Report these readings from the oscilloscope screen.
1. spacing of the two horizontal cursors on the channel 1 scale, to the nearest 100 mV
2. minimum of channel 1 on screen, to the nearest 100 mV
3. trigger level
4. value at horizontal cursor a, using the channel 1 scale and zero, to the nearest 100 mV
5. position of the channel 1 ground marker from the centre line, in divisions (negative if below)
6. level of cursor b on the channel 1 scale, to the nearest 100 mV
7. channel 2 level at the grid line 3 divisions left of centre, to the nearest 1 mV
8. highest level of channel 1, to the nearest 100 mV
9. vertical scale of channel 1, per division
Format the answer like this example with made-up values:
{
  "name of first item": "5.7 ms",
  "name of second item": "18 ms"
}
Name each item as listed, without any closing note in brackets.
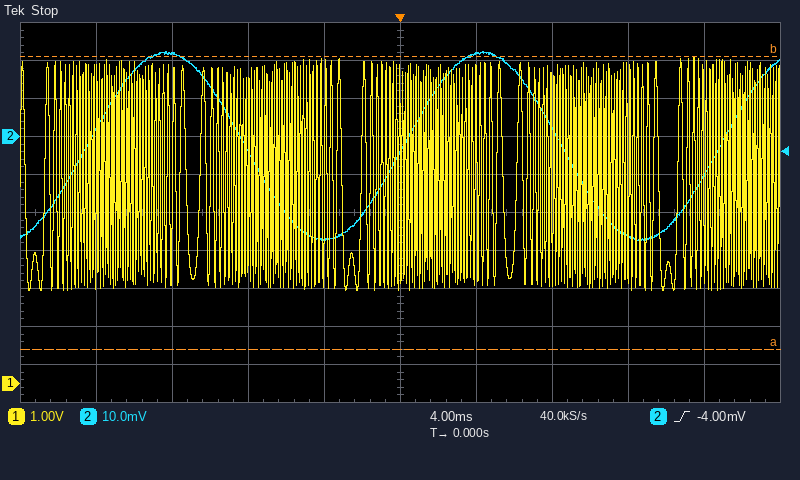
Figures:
{
  "spacing of the two horizontal cursors on the channel 1 scale, to the nearest 100 mV": "7.7 V",
  "minimum of channel 1 on screen, to the nearest 100 mV": "2.4 V",
  "trigger level": "-4.00 mV",
  "value at horizontal cursor a, using the channel 1 scale and zero, to the nearest 100 mV": "900 mV",
  "position of the channel 1 ground marker from the centre line, in divisions": "-4.5 div",
  "level of cursor b on the channel 1 scale, to the nearest 100 mV": "8.6 V",
  "channel 2 level at the grid line 3 divisions left of centre, to the nearest 1 mV": "22 mV",
  "highest level of channel 1, to the nearest 100 mV": "8.6 V",
  "vertical scale of channel 1, per division": "1 V"
}
